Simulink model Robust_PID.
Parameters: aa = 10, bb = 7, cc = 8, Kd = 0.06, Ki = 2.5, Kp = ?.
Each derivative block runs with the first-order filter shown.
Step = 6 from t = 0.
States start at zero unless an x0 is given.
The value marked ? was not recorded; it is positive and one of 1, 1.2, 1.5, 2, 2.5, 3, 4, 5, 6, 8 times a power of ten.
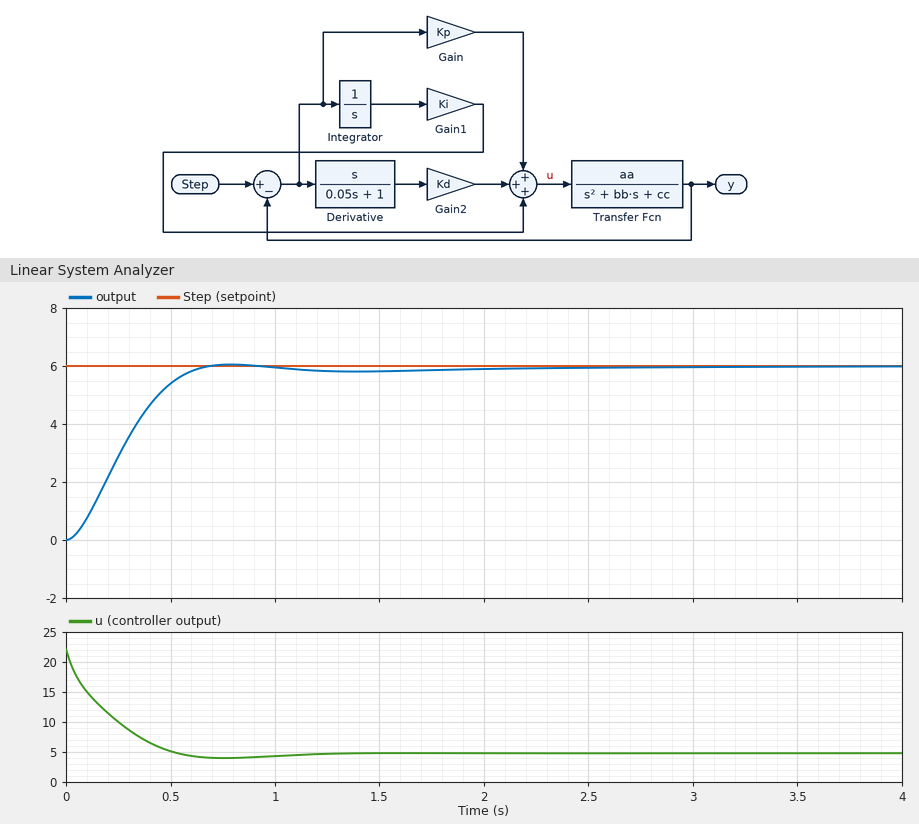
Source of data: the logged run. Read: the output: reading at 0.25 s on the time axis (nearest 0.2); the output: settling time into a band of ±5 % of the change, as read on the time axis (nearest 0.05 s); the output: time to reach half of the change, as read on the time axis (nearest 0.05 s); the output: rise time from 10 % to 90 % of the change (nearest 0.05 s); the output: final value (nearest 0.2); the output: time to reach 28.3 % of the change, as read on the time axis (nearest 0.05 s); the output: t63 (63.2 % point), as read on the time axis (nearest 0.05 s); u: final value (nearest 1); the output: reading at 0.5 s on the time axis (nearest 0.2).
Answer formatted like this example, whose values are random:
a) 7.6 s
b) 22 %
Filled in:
a) 2.8
b) 0.55 s
c) 0.25 s
d) 0.40 s
e) 6.0
f) 0.15 s
g) 0.30 s
h) 5
i) 5.4
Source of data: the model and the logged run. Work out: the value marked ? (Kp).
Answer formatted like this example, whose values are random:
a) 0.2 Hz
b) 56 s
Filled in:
a) 2.5
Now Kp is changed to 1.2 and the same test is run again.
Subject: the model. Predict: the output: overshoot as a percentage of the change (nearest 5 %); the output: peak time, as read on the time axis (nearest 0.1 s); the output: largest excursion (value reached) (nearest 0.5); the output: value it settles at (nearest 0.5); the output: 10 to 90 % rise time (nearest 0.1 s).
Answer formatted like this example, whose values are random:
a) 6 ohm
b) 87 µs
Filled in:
a) 10 %
b) 1.4 s
c) 6.5
d) 6.0
e) 0.6 s
